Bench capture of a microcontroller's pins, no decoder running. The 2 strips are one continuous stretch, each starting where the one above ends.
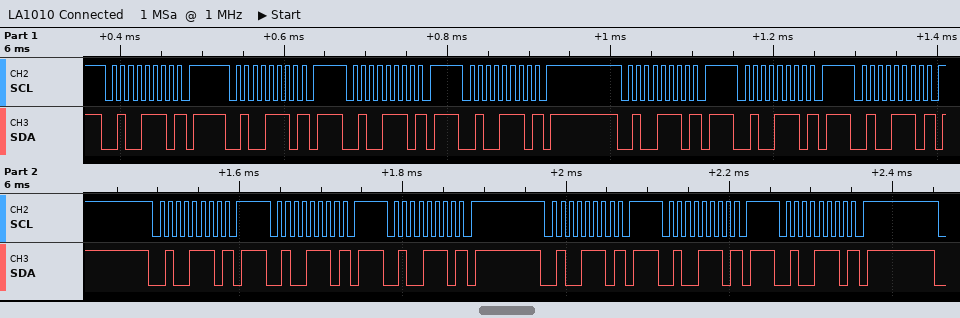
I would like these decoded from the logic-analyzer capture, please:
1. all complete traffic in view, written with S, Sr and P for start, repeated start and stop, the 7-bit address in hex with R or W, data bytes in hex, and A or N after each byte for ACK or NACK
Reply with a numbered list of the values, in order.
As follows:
1. S 27W N P S 27W N P S 27W N P S 27W N P S 27W N P S 27W N P S 27W N P S 27W N P S 27W N P S 27W N P S 27W N P S 27W N P S 27W N P
